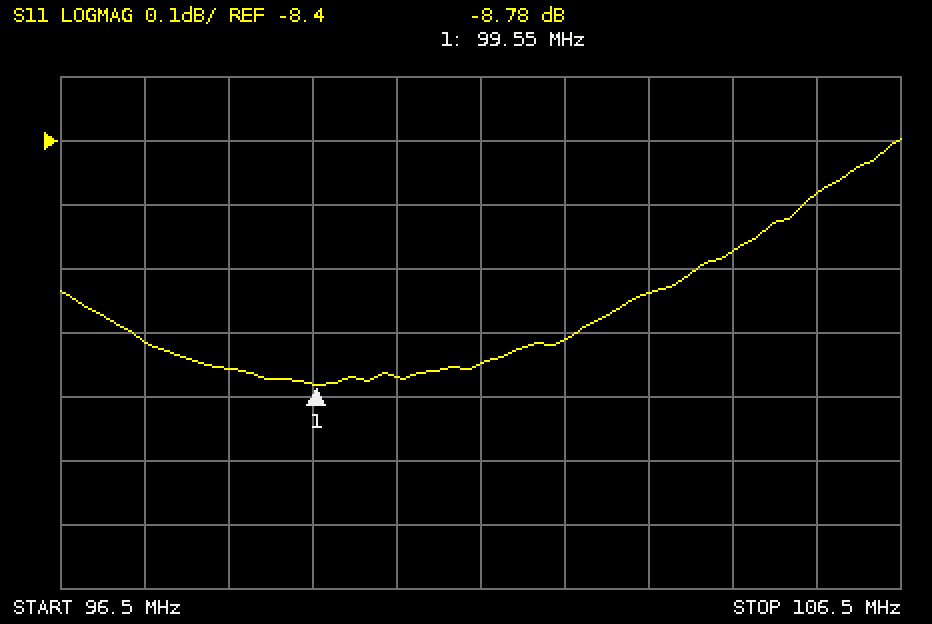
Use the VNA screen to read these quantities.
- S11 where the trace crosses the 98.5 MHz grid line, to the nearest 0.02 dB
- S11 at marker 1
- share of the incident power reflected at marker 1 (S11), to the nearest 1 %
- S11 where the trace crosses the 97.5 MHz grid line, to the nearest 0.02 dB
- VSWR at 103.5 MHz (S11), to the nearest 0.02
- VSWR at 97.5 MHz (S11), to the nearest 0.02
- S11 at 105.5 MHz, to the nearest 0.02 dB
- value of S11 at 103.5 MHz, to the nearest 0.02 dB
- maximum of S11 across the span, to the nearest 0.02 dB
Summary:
-8.76 dB
-8.78 dB
13 %
-8.72 dB
2.18
2.16
-8.48 dB
-8.64 dB
-8.40 dB
